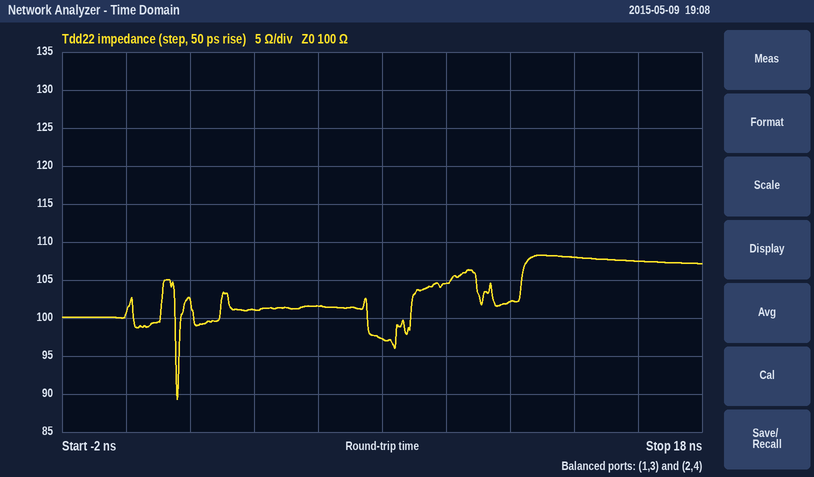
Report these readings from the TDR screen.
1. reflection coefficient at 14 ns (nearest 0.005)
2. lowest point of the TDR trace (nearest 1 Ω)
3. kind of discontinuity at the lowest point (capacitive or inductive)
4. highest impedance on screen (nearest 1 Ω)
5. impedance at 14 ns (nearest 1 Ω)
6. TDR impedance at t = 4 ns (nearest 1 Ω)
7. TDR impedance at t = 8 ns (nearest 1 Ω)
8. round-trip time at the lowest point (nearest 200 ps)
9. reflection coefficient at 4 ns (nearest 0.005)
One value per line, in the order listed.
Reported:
+0.040
89 Ω
capacitive
108 Ω
108 Ω
101 Ω
97 Ω
1.6 ns
+0.005
